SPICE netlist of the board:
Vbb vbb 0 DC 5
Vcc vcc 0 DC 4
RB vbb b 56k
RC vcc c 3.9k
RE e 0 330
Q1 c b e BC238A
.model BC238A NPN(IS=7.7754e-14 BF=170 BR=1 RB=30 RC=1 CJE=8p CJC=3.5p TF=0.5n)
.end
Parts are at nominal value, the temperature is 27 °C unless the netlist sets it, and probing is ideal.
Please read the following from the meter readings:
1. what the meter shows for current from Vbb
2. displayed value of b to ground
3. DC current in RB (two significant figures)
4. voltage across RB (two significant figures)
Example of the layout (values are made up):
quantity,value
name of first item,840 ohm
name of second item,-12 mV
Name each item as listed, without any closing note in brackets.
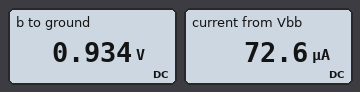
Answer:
quantity,value
what the meter shows for current from Vbb,72.6 µA
displayed value of b to ground,0.934 V
DC current in RB,73 µA
voltage across RB,4.1 V
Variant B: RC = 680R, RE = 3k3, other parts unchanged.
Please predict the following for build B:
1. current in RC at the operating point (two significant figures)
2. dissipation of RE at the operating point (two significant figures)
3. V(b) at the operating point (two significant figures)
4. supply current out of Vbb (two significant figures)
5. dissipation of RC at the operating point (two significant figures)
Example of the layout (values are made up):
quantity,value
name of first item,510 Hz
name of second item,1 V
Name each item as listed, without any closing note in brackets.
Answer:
quantity,value
current in RC at the operating point,960 µA
dissipation of RE at the operating point,3.2 mW
V(b) at the operating point,3.8 V
supply current out of Vbb,21 µA
dissipation of RC at the operating point,630 µW
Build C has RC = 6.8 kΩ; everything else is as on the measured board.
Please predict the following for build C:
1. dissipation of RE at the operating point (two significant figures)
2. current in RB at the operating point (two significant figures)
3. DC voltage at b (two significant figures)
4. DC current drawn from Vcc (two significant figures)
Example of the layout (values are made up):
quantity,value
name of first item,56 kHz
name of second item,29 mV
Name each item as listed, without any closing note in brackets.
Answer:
quantity,value
dissipation of RE at the operating point,130 µW
current in RB at the operating point,75 µA
DC voltage at b,800 mV
DC current drawn from Vcc,550 µA
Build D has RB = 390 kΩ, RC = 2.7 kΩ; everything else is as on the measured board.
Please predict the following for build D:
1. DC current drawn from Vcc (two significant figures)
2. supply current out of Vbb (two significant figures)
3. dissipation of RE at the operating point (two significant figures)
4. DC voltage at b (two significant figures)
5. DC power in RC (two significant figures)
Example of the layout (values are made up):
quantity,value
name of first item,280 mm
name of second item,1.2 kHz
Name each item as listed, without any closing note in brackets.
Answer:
quantity,value
DC current drawn from Vcc,1.3 mA
supply current out of Vbb,10 µA
dissipation of RE at the operating point,540 µW
DC voltage at b,1.0 V
DC power in RC,4.3 mW
